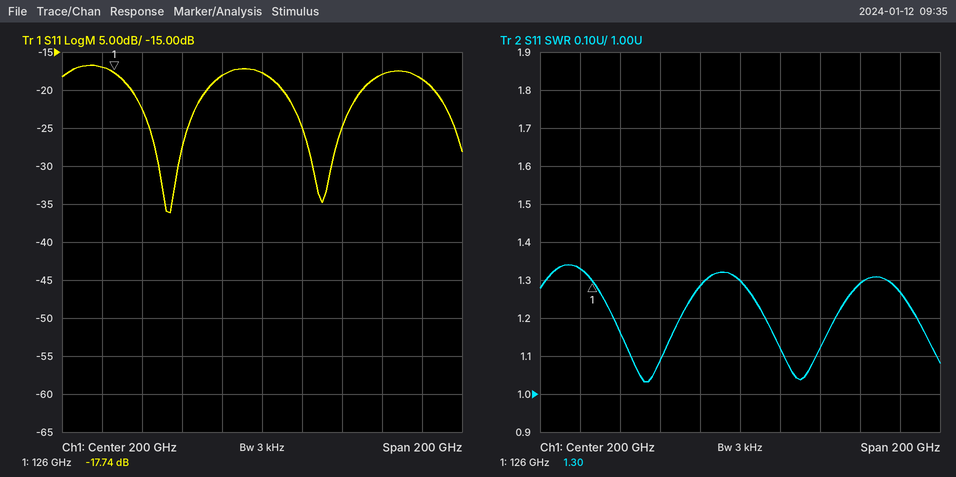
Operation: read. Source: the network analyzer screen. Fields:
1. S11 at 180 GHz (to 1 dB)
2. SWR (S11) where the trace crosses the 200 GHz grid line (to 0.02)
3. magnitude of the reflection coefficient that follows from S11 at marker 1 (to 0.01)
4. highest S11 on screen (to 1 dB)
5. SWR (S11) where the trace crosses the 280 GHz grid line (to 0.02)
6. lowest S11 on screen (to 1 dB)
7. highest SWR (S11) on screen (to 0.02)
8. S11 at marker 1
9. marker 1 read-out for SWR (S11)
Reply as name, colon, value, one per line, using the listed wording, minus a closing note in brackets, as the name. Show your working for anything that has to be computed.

S11 at 180 GHz: -18 dB
SWR (S11) where the trace crosses the 200 GHz grid line: 1.30
magnitude of the reflection coefficient that follows from S11 at marker 1: 10^(-17.74/20) ≈ 0.13
highest S11 on screen: -17 dB
SWR (S11) where the trace crosses the 280 GHz grid line: 1.26
lowest S11 on screen: -36 dB
highest SWR (S11) on screen: 1.34
S11 at marker 1: -17.74 dB
marker 1 read-out for SWR: 1.30
